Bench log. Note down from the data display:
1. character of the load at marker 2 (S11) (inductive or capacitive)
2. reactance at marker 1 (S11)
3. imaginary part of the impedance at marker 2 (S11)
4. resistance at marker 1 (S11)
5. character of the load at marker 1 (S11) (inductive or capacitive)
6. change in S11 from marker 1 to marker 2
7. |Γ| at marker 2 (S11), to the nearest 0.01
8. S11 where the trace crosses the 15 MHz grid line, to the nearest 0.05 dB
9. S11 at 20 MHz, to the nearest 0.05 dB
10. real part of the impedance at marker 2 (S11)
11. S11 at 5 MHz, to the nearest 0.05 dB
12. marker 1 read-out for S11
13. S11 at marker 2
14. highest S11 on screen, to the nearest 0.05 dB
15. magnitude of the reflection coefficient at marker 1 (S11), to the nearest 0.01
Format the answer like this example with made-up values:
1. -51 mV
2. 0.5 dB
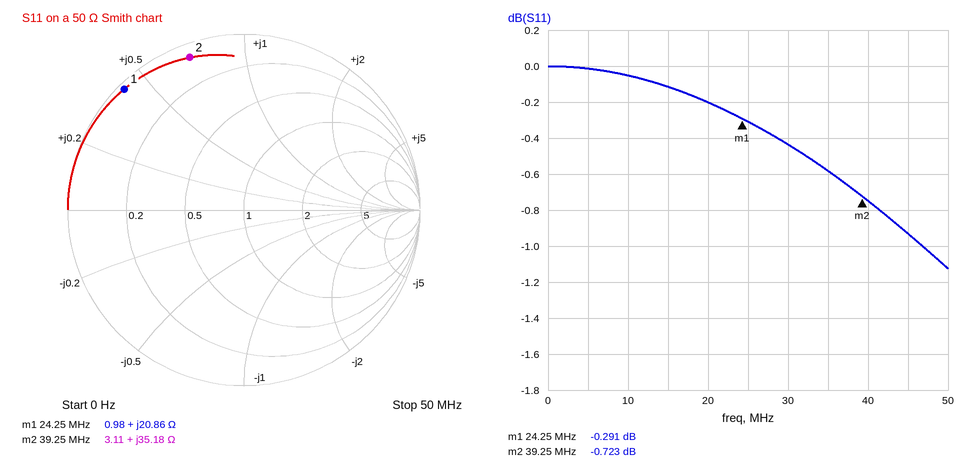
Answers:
1. inductive
2. +20.86 Ω
3. +35.18 Ω
4. 0.98 Ω
5. inductive
6. -0.432 dB
7. 0.92
8. -0.10 dB
9. -0.20 dB
10. 3.11 Ω
11. 0.00 dB
12. -0.291 dB
13. -0.723 dB
14. 0.00 dB
15. 0.97
